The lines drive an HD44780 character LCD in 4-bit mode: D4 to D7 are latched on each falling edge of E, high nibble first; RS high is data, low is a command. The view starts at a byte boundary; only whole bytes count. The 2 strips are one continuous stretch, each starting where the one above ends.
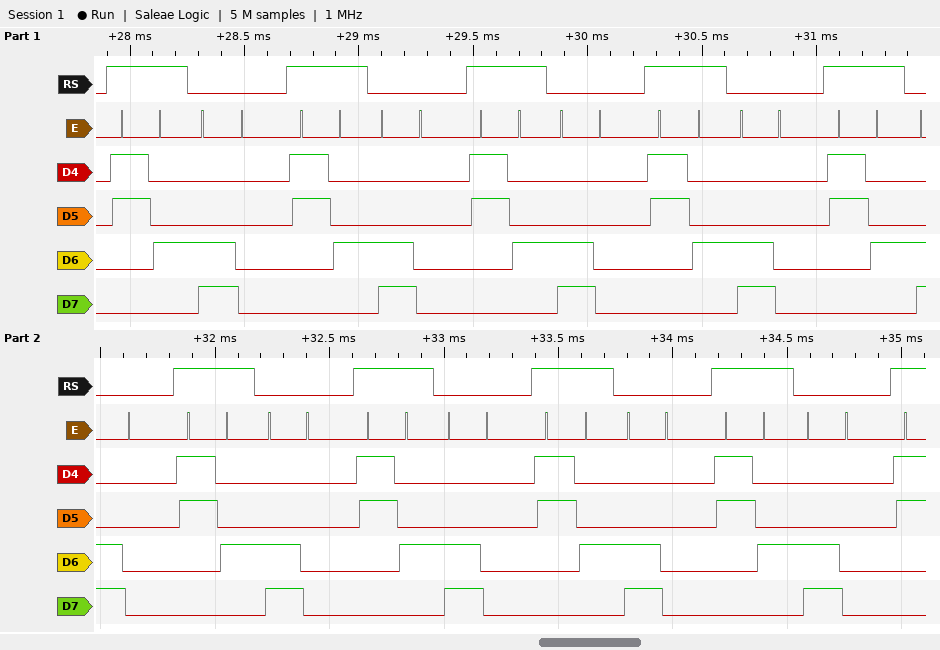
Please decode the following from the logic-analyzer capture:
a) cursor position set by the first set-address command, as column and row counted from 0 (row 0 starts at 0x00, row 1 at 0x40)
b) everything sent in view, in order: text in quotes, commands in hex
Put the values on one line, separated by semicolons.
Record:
column 0, row 1; "4" 0xC0 "4" 0xC0 "4" 0xC0 "4" 0xC0 "4" 0xC0 "4" 0xC0 "4" 0xC0 "4" 0xC0 "4" 0xC0
